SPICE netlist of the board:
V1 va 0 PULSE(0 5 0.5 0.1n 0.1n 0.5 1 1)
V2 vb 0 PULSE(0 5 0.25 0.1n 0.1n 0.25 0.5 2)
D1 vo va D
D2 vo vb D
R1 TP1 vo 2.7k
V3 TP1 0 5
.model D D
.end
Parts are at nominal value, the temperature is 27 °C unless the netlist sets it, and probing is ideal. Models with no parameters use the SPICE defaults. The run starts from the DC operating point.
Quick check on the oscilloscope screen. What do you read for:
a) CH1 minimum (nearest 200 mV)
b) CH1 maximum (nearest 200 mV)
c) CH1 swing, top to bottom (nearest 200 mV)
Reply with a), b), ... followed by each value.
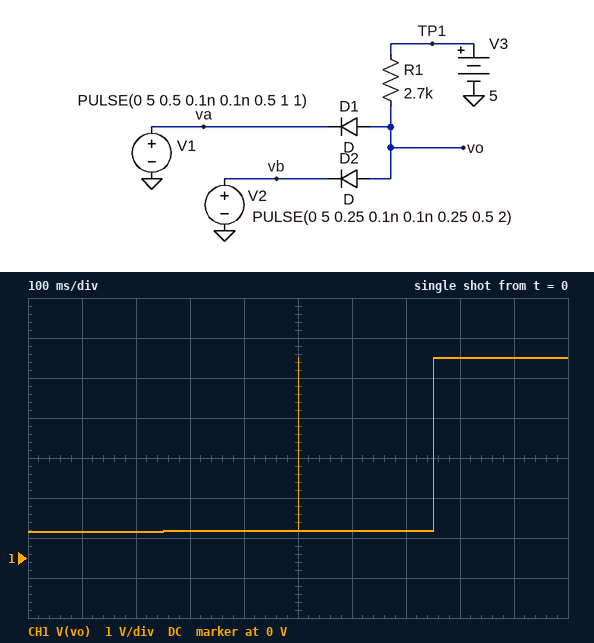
a) 600 mV
b) 5.0 V
c) 4.4 V
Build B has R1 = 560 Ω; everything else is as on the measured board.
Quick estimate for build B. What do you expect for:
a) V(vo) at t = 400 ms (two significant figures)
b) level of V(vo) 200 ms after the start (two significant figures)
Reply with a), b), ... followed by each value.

a) 710 mV
b) 690 mV
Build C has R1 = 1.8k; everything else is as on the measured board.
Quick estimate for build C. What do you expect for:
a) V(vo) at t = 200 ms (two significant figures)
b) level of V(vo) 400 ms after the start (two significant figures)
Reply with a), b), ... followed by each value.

a) 660 mV
b) 680 mV
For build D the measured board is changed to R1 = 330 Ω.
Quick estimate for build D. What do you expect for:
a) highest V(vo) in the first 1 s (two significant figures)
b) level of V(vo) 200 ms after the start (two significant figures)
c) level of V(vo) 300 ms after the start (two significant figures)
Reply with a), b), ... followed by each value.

a) 5.0 V
b) 700 mV
c) 720 mV
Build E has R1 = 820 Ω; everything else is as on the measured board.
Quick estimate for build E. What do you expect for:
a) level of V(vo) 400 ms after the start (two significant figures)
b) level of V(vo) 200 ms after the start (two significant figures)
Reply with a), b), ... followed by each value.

a) 700 mV
b) 680 mV
